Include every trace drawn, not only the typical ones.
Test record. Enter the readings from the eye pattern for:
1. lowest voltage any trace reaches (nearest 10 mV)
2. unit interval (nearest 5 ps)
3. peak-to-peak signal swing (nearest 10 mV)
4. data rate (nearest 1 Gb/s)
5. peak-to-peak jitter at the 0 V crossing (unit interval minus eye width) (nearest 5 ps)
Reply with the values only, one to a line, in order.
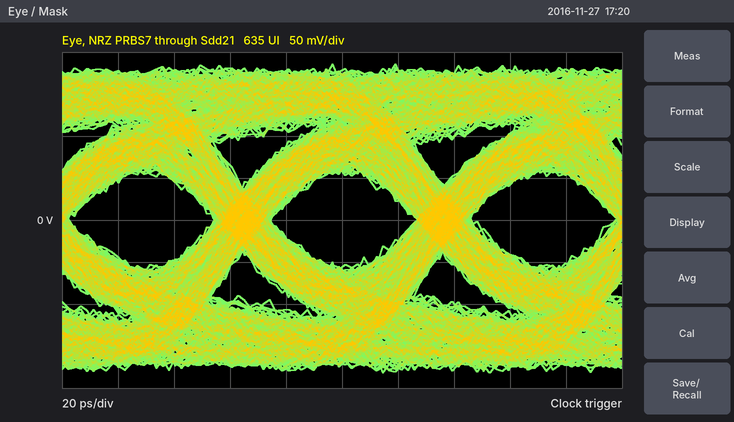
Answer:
-180 mV
70 ps
370 mV
14 Gb/s
20 ps
